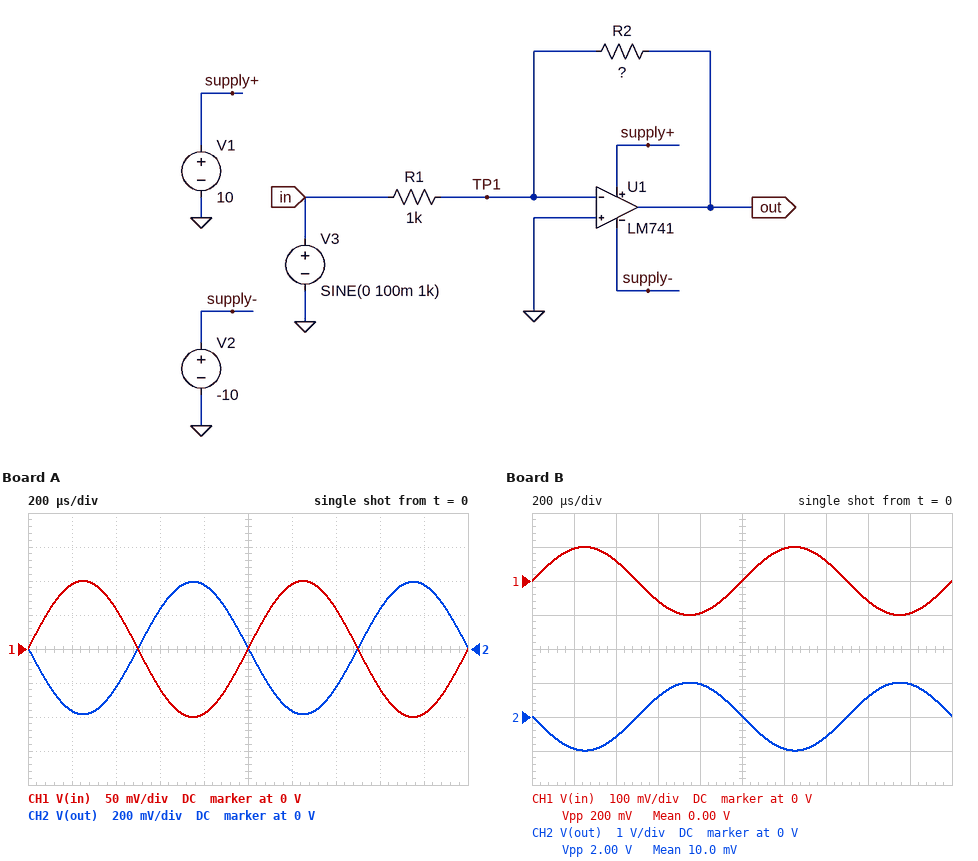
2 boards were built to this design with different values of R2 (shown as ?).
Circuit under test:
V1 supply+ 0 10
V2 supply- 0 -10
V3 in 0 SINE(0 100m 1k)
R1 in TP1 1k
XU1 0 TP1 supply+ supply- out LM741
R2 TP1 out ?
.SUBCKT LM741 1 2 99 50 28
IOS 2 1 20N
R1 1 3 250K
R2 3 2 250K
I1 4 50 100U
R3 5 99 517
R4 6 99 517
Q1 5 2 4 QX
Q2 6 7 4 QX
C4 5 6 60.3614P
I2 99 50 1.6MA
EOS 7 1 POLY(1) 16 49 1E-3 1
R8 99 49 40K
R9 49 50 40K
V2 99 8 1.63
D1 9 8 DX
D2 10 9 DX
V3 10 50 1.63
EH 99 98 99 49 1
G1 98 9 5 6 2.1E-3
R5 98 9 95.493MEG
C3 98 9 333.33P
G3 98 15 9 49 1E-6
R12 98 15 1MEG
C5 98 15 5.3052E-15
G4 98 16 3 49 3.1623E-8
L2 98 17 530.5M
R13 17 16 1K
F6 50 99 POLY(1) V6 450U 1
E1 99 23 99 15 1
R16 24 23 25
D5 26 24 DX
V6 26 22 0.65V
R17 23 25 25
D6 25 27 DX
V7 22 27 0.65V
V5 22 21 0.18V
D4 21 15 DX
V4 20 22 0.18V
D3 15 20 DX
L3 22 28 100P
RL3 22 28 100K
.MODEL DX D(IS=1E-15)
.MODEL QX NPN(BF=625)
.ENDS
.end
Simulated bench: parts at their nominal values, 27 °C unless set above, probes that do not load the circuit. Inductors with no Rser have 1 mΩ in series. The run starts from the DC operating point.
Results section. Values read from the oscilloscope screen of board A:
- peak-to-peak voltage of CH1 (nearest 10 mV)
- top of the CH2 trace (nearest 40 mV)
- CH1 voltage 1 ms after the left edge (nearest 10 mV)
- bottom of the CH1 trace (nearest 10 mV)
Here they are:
200 mV
400 mV
0 V
-100 mV
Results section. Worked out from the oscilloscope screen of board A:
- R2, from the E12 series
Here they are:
3.9 kΩ
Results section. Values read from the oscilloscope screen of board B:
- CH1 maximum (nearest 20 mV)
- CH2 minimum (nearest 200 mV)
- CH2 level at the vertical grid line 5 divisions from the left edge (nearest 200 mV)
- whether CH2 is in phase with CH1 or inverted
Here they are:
100 mV
-1.0 V
0 V
inverted
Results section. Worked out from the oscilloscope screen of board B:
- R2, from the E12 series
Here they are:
10 kΩ
